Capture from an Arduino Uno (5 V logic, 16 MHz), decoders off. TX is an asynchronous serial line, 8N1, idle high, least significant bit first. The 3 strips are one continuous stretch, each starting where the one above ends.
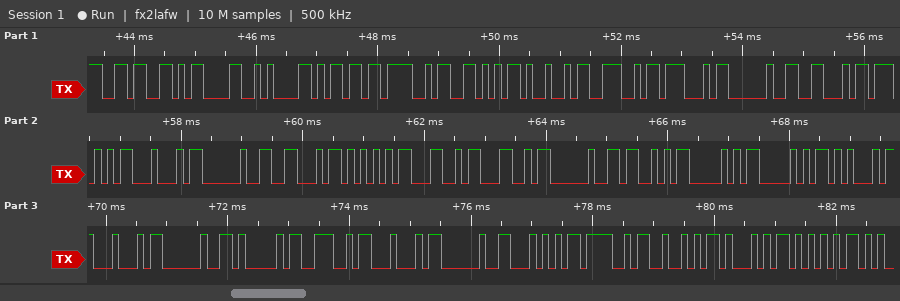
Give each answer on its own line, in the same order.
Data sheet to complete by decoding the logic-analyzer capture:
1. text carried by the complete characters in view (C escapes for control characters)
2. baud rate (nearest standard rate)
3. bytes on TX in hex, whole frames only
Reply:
"6\r\nmOVING FWD FULL SPPED AND TORQU"
9600 baud
36 0D 0A 6D 4F 56 49 4E 47 20 46 57 44 20 46 55 4C 4C 20 53 50 50 45 44 20 41 4E 44 20 54 4F 52 51 55
